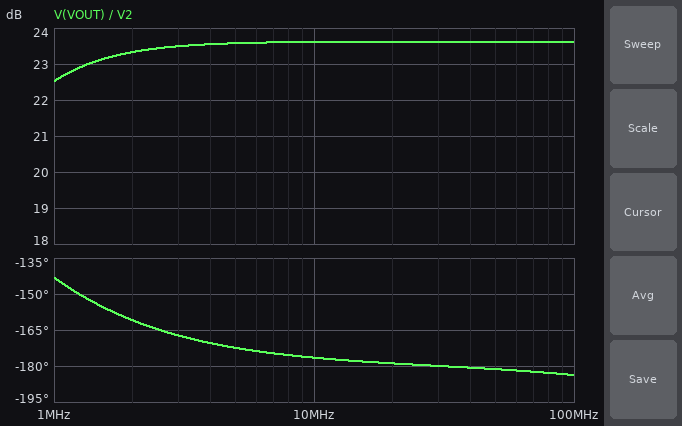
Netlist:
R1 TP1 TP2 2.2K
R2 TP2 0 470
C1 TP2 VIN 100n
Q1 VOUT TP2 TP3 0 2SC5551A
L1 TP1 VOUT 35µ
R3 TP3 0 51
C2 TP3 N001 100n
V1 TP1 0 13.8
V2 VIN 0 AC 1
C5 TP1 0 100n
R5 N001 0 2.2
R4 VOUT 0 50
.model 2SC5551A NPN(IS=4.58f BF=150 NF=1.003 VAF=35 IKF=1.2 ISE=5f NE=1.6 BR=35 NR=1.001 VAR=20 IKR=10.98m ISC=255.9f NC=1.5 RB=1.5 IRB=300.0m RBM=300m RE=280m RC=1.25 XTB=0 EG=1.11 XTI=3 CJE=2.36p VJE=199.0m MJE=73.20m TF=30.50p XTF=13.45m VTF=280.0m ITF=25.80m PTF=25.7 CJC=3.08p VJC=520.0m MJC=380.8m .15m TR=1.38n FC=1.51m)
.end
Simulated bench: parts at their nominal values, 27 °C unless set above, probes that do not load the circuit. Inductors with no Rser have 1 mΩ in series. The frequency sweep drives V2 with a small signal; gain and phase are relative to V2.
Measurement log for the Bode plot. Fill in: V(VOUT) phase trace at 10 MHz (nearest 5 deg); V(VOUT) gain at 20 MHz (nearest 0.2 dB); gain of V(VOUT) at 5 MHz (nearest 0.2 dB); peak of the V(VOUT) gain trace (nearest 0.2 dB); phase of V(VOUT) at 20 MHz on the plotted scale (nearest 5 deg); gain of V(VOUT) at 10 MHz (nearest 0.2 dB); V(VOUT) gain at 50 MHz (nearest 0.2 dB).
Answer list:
-175 deg
23.6 dB
23.6 dB
23.6 dB
-180 deg
23.6 dB
23.6 dB
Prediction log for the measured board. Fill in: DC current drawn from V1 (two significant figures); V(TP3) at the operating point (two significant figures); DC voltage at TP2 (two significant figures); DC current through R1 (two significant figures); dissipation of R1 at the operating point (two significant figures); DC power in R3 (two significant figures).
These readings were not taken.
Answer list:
310 mA
1.6 V
2.4 V
5.2 mA
59 mW
50 mW
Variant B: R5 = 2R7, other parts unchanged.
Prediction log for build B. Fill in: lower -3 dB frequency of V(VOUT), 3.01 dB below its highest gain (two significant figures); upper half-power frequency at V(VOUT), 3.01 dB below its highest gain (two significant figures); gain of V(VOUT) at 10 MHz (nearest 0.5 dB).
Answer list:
510 kHz
2.0 GHz
22.5 dB
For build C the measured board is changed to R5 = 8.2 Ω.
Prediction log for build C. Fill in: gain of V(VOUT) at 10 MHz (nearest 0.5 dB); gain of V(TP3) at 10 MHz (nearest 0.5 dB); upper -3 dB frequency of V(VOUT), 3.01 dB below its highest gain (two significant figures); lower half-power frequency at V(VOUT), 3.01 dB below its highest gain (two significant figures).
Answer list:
15.5 dB
-1.5 dB
2.7 GHz
310 kHz
